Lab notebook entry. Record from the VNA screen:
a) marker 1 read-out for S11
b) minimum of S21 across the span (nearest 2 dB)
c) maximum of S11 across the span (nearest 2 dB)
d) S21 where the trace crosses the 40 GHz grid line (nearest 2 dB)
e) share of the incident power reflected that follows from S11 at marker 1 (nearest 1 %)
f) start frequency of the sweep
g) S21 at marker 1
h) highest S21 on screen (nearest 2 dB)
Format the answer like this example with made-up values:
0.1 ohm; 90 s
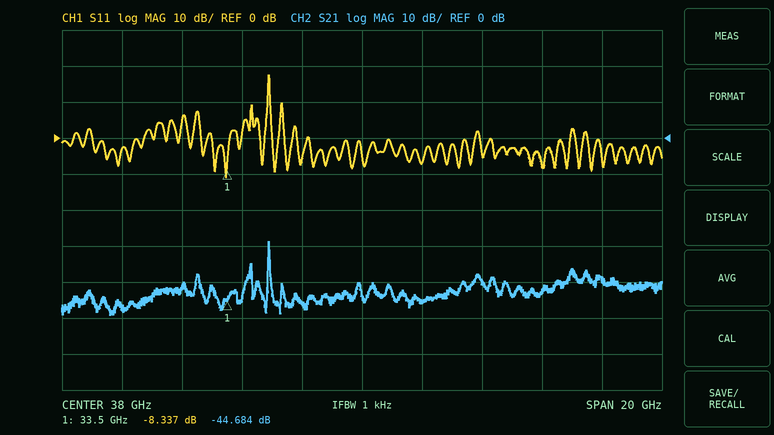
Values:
-8.337 dB; -50 dB; 18 dB; -46 dB; 15 %; 28 GHz; -44.684 dB; -28 dB
